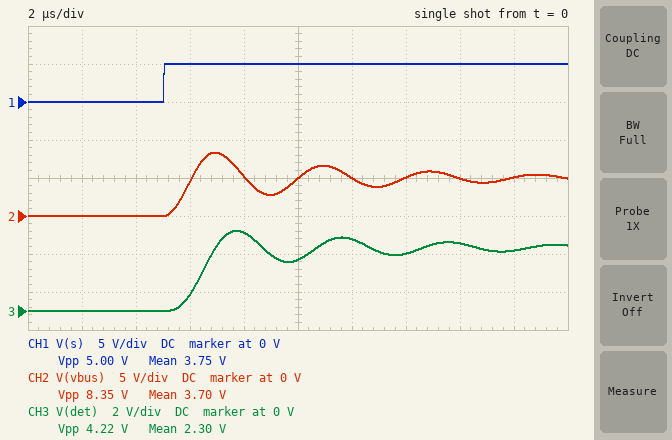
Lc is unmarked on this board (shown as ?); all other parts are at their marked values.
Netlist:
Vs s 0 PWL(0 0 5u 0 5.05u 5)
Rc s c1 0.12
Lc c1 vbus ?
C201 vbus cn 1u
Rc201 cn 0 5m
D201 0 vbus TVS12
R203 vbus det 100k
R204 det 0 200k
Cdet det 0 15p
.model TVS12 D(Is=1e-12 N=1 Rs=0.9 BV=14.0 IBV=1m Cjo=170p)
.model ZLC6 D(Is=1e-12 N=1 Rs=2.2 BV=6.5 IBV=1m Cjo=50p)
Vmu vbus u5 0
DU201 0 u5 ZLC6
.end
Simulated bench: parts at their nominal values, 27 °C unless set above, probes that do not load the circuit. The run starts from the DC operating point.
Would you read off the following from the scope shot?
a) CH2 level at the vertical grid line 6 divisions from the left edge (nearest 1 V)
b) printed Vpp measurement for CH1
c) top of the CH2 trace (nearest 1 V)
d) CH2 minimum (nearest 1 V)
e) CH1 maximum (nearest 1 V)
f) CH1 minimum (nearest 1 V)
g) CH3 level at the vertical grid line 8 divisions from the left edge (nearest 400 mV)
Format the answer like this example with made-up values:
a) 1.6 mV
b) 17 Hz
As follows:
a) 5 V
b) 5.00 V
c) 8 V
d) 0 V
e) 5 V
f) 0 V
g) 3.6 V
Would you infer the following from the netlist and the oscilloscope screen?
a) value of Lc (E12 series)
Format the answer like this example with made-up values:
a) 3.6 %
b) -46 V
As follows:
a) 390 nH
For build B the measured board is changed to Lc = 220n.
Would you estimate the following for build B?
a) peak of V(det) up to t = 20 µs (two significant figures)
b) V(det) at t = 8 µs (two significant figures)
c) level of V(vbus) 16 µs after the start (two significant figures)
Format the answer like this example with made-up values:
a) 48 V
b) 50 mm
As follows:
a) 3.7 V
b) 3.1 V
c) 5.1 V
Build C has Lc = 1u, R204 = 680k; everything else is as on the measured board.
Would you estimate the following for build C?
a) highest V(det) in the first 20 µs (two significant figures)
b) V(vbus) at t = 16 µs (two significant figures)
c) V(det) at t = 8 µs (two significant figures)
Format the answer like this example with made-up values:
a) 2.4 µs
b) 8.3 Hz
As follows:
a) 6.0 V
b) 5.2 V
c) 4.8 V
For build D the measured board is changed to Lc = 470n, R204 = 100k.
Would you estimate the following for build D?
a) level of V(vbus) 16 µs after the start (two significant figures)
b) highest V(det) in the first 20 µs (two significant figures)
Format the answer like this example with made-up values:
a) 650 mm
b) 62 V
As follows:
a) 5.9 V
b) 3.5 V
